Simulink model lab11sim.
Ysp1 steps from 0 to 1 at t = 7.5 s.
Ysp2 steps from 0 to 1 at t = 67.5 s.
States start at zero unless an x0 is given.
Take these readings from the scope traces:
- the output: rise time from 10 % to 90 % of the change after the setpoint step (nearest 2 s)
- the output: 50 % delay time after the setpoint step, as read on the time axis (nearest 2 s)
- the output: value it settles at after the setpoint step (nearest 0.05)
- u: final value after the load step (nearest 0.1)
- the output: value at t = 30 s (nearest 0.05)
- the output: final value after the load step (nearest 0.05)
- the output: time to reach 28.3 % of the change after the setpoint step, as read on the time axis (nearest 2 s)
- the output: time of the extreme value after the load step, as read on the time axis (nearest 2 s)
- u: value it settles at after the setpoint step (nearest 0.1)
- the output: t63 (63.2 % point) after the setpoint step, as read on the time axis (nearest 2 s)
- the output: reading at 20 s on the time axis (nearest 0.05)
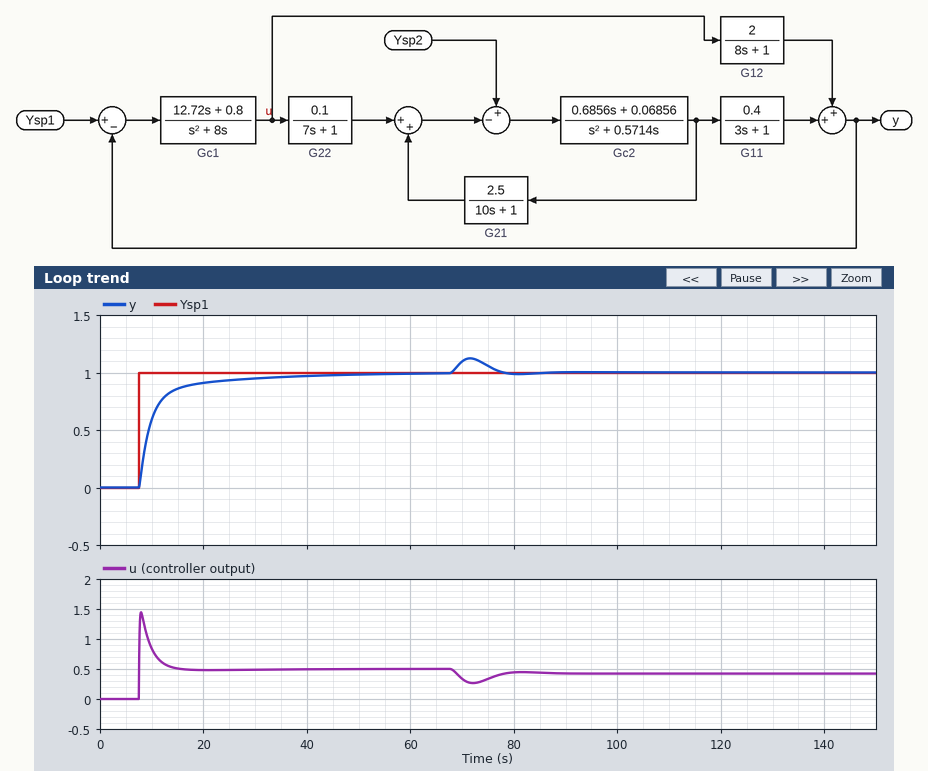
10 s
10 s
1.00
0.4
0.95
1.00
8 s
72 s
0.5
10 s
0.90
